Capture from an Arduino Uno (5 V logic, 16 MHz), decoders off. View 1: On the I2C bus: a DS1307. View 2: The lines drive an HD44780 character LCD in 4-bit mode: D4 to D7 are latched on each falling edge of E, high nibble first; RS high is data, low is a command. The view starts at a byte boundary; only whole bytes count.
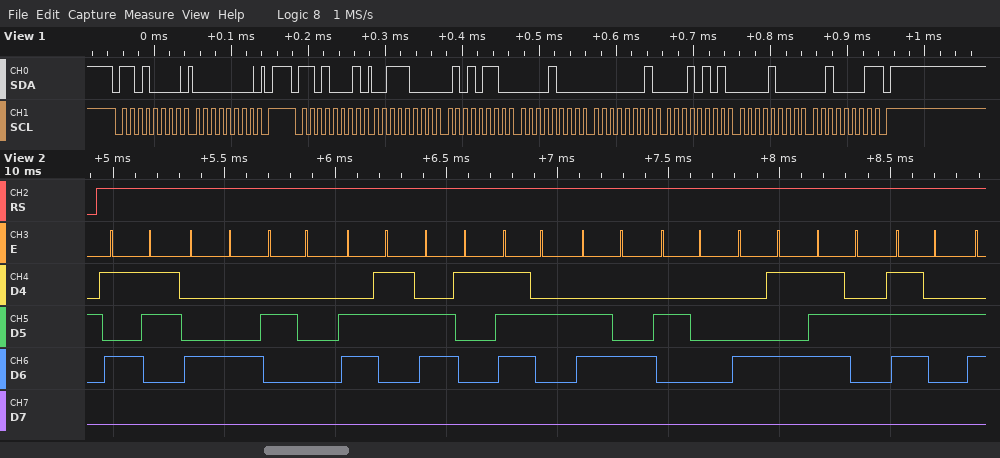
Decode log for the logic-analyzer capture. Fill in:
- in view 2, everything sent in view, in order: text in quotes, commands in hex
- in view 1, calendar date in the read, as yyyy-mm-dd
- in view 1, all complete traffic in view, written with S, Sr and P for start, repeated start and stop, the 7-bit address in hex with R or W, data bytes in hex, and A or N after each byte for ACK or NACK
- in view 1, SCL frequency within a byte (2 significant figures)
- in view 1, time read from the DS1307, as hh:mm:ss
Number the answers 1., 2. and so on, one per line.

1. "SD card Err"
2. 2021-08-15
3. S 68W A 00 A P S 68R A 38 A 56 A 08 A 01 A 15 A 08 A 21 N P
4. 100 kHz
5. 08:56:38
